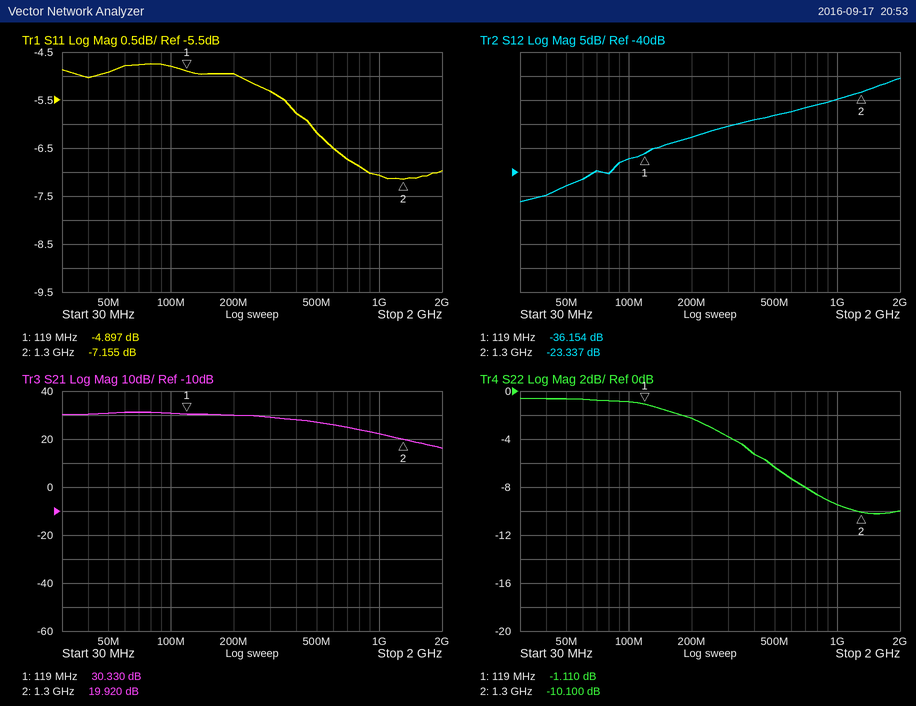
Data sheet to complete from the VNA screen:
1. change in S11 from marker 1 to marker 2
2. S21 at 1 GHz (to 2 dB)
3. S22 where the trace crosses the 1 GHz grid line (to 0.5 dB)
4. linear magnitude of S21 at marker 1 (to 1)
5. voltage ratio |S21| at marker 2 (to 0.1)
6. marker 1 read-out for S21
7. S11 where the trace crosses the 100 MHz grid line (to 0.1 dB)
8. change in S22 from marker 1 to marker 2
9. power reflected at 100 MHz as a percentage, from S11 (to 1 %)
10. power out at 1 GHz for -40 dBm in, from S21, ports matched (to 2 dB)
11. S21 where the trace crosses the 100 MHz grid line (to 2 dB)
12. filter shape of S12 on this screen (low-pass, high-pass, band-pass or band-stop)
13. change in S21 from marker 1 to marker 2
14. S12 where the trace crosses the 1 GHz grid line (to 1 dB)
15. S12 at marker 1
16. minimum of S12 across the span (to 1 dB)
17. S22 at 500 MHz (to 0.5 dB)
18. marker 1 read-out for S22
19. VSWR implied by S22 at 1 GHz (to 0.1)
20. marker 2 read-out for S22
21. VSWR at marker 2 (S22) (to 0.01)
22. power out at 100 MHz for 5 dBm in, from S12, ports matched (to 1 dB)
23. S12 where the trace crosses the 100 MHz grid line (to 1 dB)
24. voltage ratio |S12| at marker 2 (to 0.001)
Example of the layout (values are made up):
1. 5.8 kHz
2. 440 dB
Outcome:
1. -2.258 dB
2. 22 dB
3. -9.5 dB
4. 33
5. 9.9
6. 30.330 dB
7. -4.8 dB
8. -8.990 dB
9. 33 %
10. -18 dBm
11. 30 dB
12. high-pass
13. -10.410 dB
14. -25 dB
15. -36.154 dB
16. -46 dB
17. -6.5 dB
18. -1.110 dB
19. 2.0
20. -10.100 dB
21. 1.91
22. -32 dBm
23. -37 dB
24. 0.068
